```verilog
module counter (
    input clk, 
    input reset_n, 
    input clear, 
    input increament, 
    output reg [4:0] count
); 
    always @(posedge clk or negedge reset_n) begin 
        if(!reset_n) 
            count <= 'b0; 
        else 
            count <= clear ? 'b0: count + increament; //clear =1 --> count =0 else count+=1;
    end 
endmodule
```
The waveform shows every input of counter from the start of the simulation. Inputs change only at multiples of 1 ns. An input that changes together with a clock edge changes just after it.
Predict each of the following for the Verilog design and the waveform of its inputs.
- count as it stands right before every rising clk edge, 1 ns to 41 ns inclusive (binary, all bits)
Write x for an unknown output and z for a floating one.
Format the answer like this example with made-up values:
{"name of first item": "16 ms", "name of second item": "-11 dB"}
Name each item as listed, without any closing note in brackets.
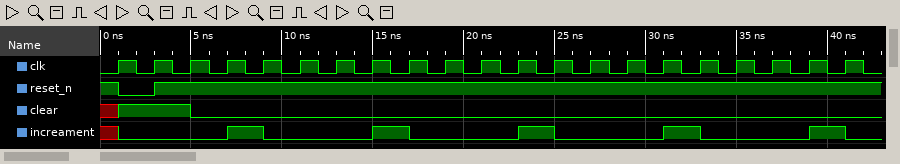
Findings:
{"count as it stands right before every rising clk edge, 1 ns to 41 ns inclusive": "x, 00000, 00000, 00000, 00000, 00001, 00001, 00001, 00001, 00010, 00010, 00010, 00010, 00011, 00011, 00011, 00011, 00100, 00100, 00100, 00100"}
